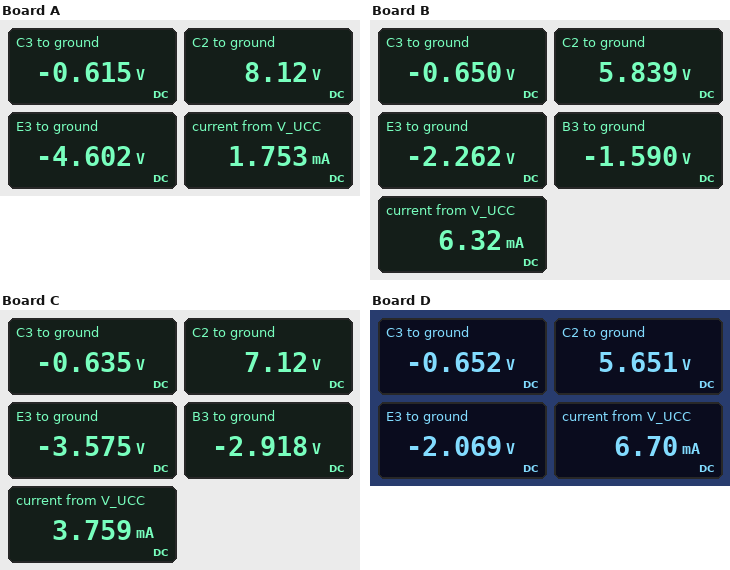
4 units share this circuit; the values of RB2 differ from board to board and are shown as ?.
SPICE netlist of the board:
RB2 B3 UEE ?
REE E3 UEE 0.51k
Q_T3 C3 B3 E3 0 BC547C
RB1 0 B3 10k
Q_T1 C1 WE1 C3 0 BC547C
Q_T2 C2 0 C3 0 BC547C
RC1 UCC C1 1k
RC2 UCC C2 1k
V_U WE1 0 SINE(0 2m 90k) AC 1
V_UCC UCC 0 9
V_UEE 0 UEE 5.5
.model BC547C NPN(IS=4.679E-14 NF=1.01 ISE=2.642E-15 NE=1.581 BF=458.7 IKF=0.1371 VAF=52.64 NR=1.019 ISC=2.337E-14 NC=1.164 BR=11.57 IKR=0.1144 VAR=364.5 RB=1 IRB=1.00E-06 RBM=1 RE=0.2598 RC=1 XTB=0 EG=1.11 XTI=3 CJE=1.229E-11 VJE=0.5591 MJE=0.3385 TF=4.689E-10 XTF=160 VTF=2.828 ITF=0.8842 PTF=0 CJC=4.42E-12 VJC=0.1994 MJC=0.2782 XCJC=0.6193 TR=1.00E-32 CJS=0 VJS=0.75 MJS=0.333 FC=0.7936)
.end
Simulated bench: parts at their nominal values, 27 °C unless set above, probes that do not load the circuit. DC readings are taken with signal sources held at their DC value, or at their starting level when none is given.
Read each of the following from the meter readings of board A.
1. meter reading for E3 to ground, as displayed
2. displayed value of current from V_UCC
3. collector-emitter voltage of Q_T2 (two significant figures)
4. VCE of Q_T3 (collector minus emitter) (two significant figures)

-4.602 V
1.753 mA
8.7 V
4.0 V
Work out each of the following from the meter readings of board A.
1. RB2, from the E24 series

3.9 kΩ
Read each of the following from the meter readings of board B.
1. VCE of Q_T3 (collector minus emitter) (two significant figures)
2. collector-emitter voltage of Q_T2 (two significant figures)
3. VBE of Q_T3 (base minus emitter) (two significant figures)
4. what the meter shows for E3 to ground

1.6 V
6.5 V
670 mV
-2.262 V
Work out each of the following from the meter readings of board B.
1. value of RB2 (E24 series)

27 kΩ
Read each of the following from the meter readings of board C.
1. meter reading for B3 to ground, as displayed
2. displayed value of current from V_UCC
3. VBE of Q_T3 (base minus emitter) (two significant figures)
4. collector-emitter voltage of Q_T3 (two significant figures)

-2.918 V
3.759 mA
660 mV
2.9 V
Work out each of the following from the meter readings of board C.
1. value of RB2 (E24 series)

9.1 kΩ
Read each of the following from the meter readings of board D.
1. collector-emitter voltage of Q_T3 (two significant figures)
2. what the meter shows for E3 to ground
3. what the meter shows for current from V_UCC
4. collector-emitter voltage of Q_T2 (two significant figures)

1.4 V
-2.069 V
6.70 mA
6.3 V
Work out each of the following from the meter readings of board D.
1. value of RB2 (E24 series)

33 kΩ
